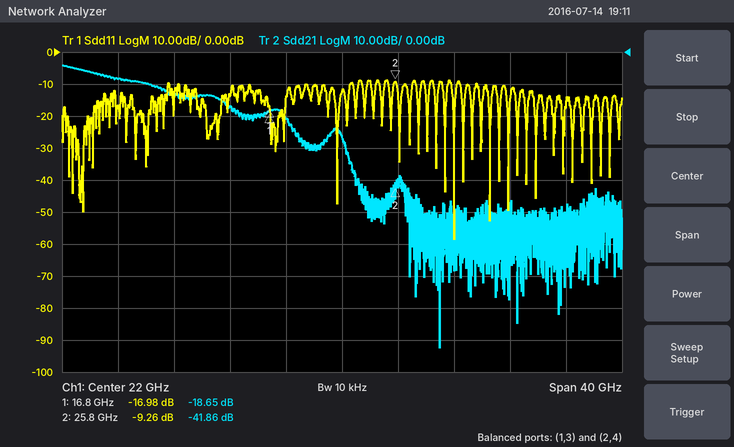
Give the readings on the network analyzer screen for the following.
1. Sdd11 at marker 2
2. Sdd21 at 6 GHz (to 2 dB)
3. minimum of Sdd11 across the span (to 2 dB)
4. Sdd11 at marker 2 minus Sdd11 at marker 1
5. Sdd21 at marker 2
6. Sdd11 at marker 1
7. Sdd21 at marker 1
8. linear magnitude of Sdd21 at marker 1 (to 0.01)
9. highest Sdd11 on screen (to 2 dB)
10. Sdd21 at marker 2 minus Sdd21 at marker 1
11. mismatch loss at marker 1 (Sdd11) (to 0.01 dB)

-9.26 dB
-8 dB
-58 dB
7.72 dB
-41.86 dB
-16.98 dB
-18.65 dB
0.12
-8 dB
-23.21 dB
0.09 dB
